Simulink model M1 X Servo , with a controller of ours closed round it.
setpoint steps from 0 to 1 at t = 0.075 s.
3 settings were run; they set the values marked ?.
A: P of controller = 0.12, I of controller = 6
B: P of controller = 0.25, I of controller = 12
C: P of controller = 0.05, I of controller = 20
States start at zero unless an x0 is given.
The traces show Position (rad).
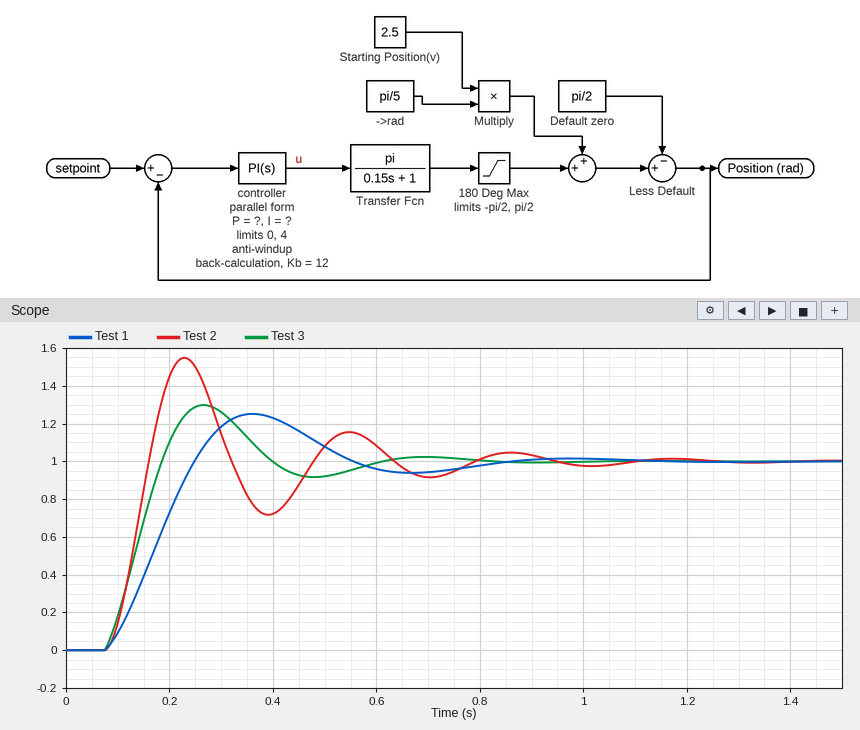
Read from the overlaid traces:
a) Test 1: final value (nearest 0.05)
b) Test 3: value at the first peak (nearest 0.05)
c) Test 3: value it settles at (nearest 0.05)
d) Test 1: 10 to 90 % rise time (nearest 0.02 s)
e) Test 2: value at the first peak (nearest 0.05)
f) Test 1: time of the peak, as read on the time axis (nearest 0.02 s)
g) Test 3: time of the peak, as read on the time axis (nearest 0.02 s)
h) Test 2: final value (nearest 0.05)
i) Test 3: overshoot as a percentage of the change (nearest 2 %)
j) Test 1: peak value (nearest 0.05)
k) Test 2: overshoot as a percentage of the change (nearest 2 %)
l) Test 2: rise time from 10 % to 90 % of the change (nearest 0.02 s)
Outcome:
1.00
1.30
1.00
0.12 s
1.55
0.36 s
0.26 s
1.00
30 %
1.25
54 %
0.06 s
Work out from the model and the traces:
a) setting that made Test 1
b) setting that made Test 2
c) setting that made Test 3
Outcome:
A
C
B
